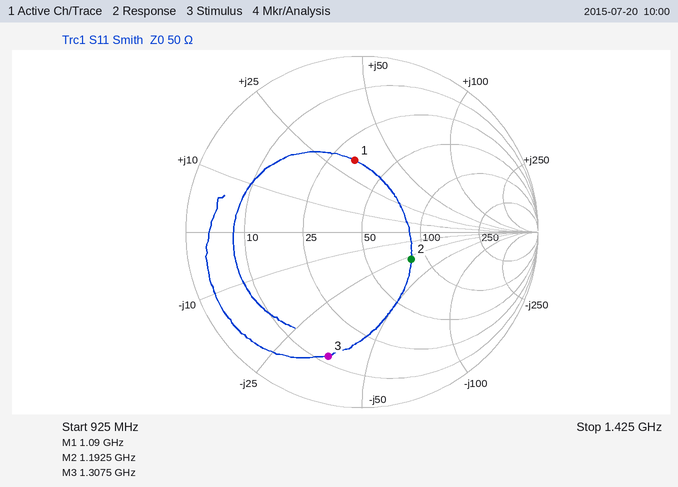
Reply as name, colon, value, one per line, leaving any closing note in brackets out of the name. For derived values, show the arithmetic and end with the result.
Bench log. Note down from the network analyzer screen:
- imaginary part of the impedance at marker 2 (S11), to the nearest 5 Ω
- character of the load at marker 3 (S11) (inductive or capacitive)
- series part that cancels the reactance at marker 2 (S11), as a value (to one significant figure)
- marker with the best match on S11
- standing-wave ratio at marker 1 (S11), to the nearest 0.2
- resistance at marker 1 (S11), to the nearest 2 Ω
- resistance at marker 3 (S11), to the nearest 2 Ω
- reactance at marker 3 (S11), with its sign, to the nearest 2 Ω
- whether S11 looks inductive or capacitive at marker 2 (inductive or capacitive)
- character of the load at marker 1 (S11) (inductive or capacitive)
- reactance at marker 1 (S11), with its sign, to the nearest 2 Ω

imaginary part of the impedance at marker 2 (S11), to the nearest 5 Ω: -30 Ω
character of the load at marker 3 (S11): capacitive
series part that cancels the reactance at marker 2 (S11), as a value: L = 30 Ω/(2π × 1.1925 GHz) ≈ 4 nH
marker with the best match on S11: marker 2
standing-wave ratio at marker 1 (S11), to the nearest 0.2: 2.4
resistance at marker 1 (S11), to the nearest 2 Ω: 34 Ω
resistance at marker 3 (S11), to the nearest 2 Ω: 12 Ω
reactance at marker 3 (S11), with its sign, to the nearest 2 Ω: -36 Ω
whether S11 looks inductive or capacitive at marker 2: capacitive
character of the load at marker 1 (S11): inductive
reactance at marker 1 (S11), with its sign, to the nearest 2 Ω: +32 Ω
